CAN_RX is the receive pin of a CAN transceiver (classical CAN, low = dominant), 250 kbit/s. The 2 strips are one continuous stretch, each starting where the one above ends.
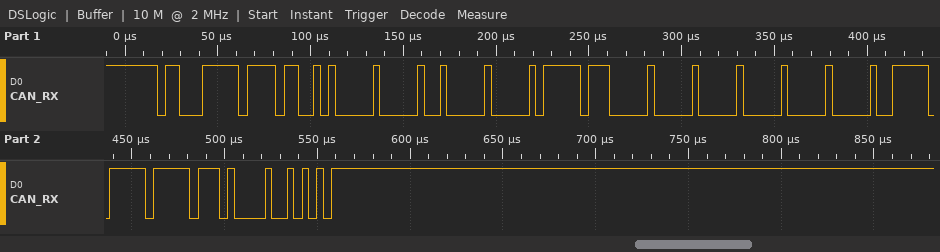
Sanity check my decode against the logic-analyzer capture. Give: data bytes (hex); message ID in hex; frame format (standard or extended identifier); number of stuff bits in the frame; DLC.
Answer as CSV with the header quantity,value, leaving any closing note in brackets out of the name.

quantity,value
data bytes,00 FF 00 00 00 00 FF FF
message ID in hex,0x18FECA00
frame format,extended
number of stuff bits in the frame,15
DLC,8
